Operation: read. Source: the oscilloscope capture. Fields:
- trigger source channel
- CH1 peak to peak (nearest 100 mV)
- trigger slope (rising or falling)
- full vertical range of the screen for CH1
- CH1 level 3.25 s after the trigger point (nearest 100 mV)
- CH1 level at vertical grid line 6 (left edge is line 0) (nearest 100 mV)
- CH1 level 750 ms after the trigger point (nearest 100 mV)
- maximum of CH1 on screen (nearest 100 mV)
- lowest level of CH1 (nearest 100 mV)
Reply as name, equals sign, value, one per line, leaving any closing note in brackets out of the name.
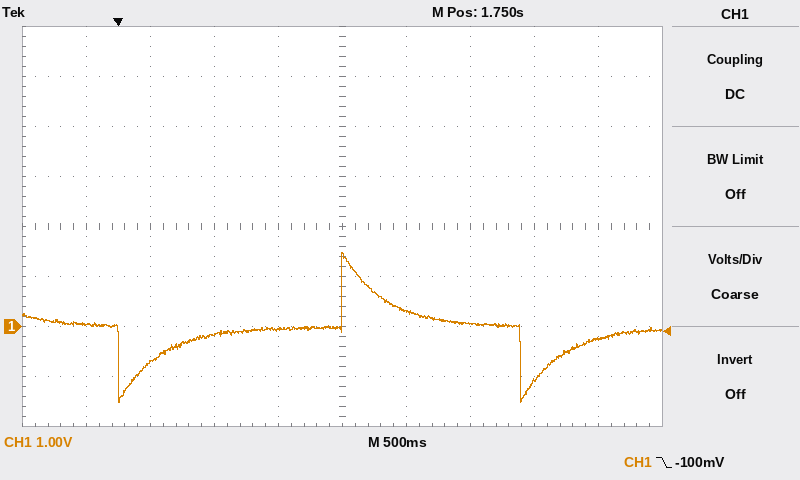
trigger source channel = CH1
CH1 peak to peak = 3.0 V
trigger slope = falling
full vertical range of the screen for CH1 = 8 V
CH1 level 3.25 s after the trigger point = -1.1 V
CH1 level at vertical grid line 6 (left edge is line 0) = 300 mV
CH1 level 750 ms after the trigger point = -200 mV
maximum of CH1 on screen = 1.5 V
lowest level of CH1 = -1.5 V
